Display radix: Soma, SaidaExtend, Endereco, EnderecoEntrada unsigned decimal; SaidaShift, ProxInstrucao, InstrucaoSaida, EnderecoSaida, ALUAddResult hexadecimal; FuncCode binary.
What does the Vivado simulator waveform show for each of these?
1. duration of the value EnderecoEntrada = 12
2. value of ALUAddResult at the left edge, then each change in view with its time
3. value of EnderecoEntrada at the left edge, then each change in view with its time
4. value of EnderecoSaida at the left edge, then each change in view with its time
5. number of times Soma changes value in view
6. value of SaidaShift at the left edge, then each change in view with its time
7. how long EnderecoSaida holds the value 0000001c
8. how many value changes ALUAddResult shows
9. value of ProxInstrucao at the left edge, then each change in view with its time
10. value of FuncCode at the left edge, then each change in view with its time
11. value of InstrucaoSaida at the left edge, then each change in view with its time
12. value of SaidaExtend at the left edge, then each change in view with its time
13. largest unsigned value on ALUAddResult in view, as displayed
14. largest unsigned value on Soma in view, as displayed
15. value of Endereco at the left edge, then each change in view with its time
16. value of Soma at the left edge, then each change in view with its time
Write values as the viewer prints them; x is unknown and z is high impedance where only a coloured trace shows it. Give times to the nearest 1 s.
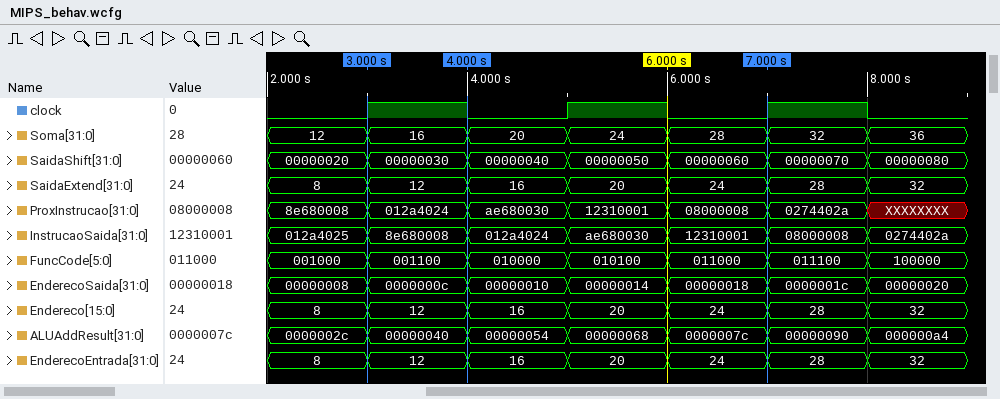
1 s
0000002c, 00000040 at 3 s, 00000054 at 4 s, 00000068 at 5 s, 0000007c at 6 s, 00000090 at 7 s, 000000a4 at 8 s
8, 12 at 3 s, 16 at 4 s, 20 at 5 s, 24 at 6 s, 28 at 7 s, 32 at 8 s
00000008, 0000000c at 3 s, 00000010 at 4 s, 00000014 at 5 s, 00000018 at 6 s, 0000001c at 7 s, 00000020 at 8 s
6
00000020, 00000030 at 3 s, 00000040 at 4 s, 00000050 at 5 s, 00000060 at 6 s, 00000070 at 7 s, 00000080 at 8 s
1 s
6
8e680008, 012a4024 at 3 s, ae680030 at 4 s, 12310001 at 5 s, 08000008 at 6 s, 0274402a at 7 s, XXXXXXXX at 8 s
001000, 001100 at 3 s, 010000 at 4 s, 010100 at 5 s, 011000 at 6 s, 011100 at 7 s, 100000 at 8 s
012a4025, 8e680008 at 3 s, 012a4024 at 4 s, ae680030 at 5 s, 12310001 at 6 s, 08000008 at 7 s, 0274402a at 8 s
8, 12 at 3 s, 16 at 4 s, 20 at 5 s, 24 at 6 s, 28 at 7 s, 32 at 8 s
000000a4
36
8, 12 at 3 s, 16 at 4 s, 20 at 5 s, 24 at 6 s, 28 at 7 s, 32 at 8 s
12, 16 at 3 s, 20 at 4 s, 24 at 5 s, 28 at 6 s, 32 at 7 s, 36 at 8 s
